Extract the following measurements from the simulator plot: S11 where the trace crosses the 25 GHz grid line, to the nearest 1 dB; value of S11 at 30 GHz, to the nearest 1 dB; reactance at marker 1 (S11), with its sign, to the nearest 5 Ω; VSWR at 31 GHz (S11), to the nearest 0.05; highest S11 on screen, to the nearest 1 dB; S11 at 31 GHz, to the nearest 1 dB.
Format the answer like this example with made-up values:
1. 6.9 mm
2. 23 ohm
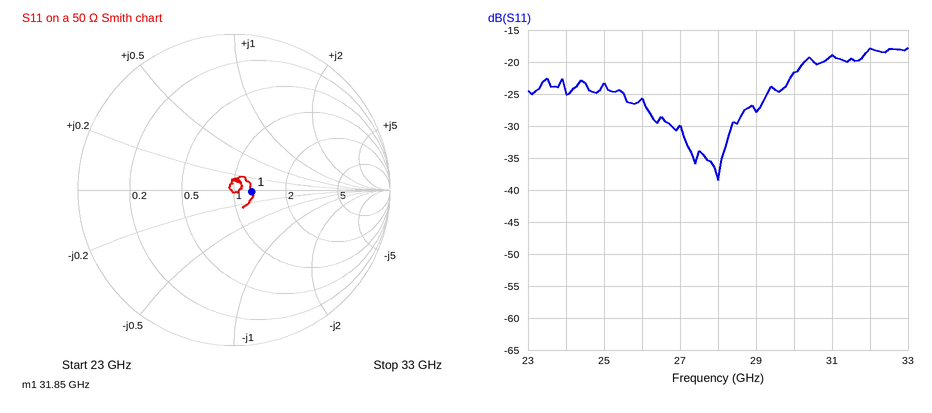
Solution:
1. -23 dB
2. -22 dB
3. 0 Ω
4. 1.25
5. -18 dB
6. -19 dB
